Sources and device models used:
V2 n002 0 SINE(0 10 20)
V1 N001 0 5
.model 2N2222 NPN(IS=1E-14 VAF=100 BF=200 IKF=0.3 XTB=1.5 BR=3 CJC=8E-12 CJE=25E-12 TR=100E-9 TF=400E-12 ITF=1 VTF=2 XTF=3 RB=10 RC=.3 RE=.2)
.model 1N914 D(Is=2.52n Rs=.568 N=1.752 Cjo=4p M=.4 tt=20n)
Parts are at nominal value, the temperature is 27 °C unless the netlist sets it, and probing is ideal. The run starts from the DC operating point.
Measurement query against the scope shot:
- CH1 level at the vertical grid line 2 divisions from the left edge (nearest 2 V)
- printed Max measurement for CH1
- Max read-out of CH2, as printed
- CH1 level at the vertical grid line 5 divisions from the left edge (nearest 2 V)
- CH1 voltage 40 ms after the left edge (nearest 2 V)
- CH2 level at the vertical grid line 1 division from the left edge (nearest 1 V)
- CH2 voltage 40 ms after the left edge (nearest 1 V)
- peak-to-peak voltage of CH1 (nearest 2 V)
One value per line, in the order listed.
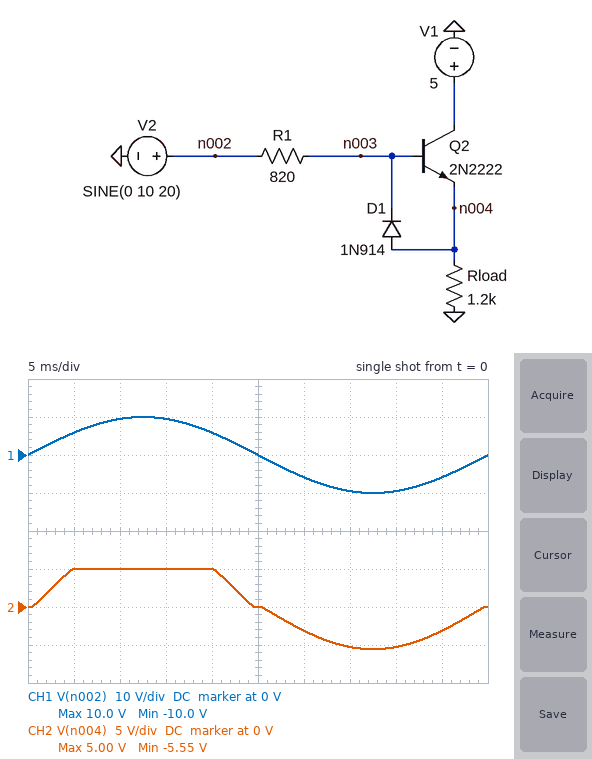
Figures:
10 V
10.0 V
5.00 V
0 V
-10 V
5 V
-5 V
20 V
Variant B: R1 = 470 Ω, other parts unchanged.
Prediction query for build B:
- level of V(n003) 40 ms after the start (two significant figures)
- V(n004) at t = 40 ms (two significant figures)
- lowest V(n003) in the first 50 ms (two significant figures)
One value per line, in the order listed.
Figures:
-7.0 V
-6.4 V
-7.4 V
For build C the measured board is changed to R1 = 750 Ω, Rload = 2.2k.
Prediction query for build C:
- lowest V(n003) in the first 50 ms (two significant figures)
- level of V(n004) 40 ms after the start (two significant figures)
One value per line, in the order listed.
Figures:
-7.6 V
-6.6 V
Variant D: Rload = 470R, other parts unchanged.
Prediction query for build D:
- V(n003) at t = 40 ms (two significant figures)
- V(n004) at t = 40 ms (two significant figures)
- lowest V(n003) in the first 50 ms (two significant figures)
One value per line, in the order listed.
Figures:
-3.9 V
-3.2 V
-4.1 V
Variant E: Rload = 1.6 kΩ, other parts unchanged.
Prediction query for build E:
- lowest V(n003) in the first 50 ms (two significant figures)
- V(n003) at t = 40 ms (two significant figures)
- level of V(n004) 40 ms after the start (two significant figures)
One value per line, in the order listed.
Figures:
-6.8 V
-6.5 V
-5.9 V
